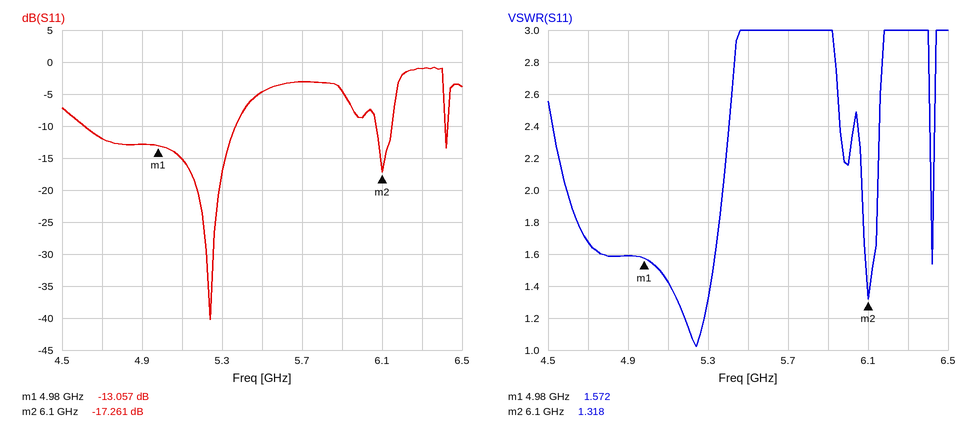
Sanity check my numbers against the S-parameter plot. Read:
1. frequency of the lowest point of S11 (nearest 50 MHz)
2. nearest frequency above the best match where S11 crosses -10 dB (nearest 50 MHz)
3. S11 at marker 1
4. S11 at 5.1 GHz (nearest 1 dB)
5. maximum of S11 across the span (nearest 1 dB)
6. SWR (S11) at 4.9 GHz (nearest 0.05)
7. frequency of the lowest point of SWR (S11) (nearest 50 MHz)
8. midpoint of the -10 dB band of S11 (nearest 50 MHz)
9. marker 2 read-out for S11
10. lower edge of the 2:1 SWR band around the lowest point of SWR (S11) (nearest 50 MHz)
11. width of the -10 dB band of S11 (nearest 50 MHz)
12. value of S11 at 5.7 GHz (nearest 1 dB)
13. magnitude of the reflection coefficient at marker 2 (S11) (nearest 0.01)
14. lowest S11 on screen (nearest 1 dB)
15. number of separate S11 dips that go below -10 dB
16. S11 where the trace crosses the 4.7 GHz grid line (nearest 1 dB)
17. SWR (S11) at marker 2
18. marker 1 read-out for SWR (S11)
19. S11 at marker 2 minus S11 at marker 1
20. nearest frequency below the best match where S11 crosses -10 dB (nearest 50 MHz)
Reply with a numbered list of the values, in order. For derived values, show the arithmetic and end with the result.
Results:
1. 5.25 GHz
2. 5.35 GHz
3. -13.057 dB
4. -15 dB
5. -1 dB
6. 1.60
7. 5.25 GHz
8. 5.00 GHz
9. -17.261 dB
10. 4.60 GHz
11. 5.35 GHz − 4.60 GHz = 750 MHz
12. -3 dB
13. 10^(-17.261/20) ≈ 0.14
14. -40 dB
15. 3
16. -12 dB
17. 1.318
18. 1.572
19. -17.261 − (-13.057) = -4.204 dB
20. 4.60 GHz
